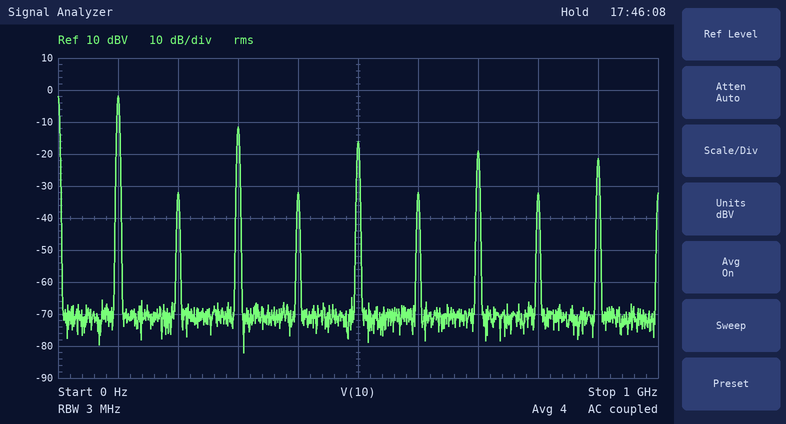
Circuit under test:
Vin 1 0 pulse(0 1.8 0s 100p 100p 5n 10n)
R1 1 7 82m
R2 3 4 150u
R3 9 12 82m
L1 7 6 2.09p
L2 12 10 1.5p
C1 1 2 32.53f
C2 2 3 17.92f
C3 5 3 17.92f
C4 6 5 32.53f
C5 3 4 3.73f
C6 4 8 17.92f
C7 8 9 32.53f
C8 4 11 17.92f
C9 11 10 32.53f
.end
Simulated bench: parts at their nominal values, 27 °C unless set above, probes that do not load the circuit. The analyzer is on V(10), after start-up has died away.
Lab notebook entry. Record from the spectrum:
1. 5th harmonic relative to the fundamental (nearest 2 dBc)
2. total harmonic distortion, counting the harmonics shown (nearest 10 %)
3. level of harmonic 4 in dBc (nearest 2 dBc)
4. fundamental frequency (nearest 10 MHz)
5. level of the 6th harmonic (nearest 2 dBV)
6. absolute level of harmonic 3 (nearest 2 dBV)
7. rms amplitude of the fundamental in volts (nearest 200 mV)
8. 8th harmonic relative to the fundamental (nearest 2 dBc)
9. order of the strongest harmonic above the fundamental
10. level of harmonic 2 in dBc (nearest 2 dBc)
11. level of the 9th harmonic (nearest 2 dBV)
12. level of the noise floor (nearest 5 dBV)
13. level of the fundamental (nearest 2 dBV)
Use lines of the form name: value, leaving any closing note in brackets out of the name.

5th harmonic relative to the fundamental: -14 dBc
total harmonic distortion, counting the harmonics shown: 40 %
level of harmonic 4 in dBc: -30 dBc
fundamental frequency: 100 MHz
level of the 6th harmonic: -32 dBV
absolute level of harmonic 3: -12 dBV
rms amplitude of the fundamental in volts: 800 mV
8th harmonic relative to the fundamental: -30 dBc
order of the strongest harmonic above the fundamental: 3
level of harmonic 2 in dBc: -30 dBc
level of the 9th harmonic: -22 dBV
level of the noise floor: -70 dBV
level of the fundamental: -2 dBV
